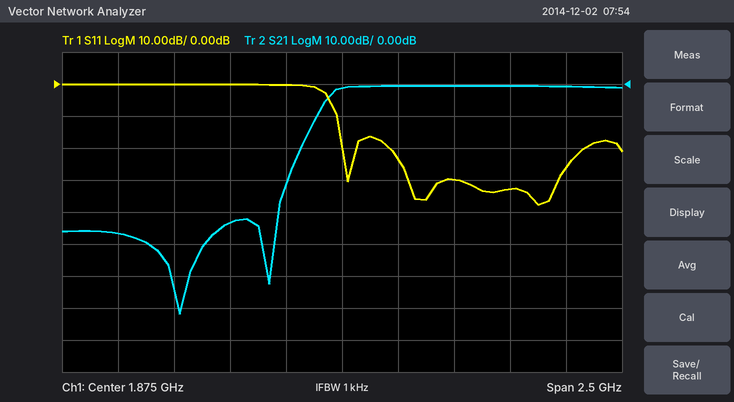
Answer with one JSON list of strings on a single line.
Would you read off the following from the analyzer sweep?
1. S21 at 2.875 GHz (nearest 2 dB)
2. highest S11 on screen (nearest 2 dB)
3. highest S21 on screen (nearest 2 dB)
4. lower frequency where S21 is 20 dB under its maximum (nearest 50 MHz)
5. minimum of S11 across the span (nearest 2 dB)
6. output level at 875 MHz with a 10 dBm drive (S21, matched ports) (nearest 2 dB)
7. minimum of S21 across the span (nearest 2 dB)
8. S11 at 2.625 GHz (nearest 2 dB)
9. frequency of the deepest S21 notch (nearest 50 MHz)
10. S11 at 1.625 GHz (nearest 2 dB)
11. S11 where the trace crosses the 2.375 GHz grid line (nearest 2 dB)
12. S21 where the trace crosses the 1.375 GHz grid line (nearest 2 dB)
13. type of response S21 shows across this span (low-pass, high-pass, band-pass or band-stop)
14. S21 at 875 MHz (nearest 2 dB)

["0 dB", "0 dB", "0 dB", "1.70 GHz", "-38 dB", "-36 dBm", "-72 dB", "-32 dB", "1.15 GHz", "0 dB", "-30 dB", "-44 dB", "high-pass", "-46 dB"]
